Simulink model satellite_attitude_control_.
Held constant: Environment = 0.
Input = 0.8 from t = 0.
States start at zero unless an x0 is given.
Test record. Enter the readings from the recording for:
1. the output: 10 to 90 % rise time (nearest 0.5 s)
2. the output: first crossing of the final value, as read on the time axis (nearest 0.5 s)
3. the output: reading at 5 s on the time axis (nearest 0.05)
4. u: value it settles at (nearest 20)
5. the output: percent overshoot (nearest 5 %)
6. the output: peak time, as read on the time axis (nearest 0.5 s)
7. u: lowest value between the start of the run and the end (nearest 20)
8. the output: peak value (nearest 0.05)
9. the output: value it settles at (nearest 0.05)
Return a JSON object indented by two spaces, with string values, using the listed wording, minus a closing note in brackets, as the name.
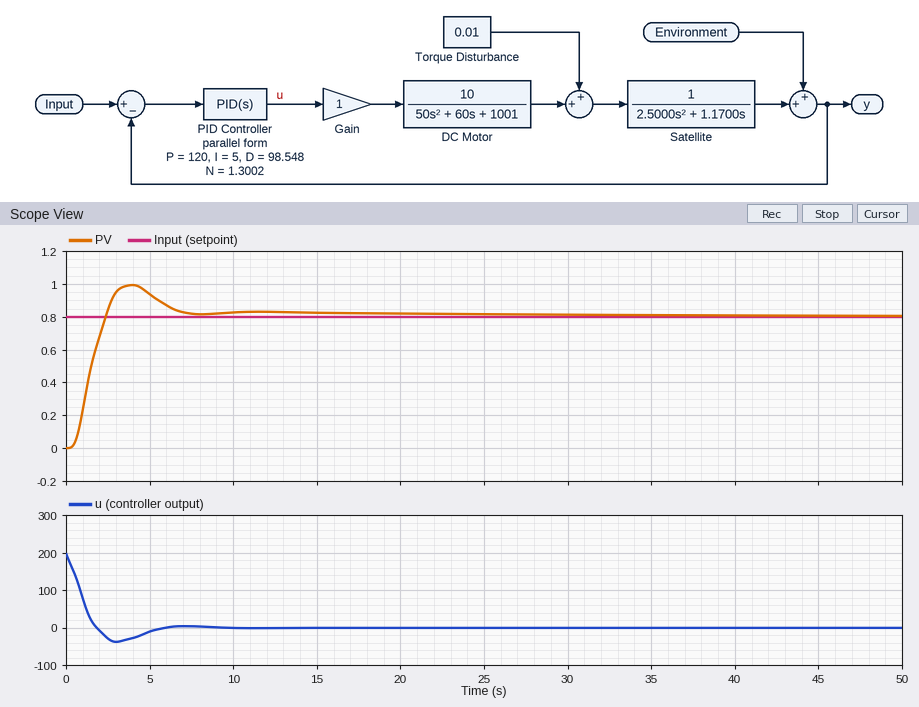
{
  "the output: 10 to 90 % rise time": "1.5 s",
  "the output: first crossing of the final value, as read on the time axis": "2.5 s",
  "the output: reading at 5 s on the time axis": "0.95",
  "u: value it settles at": "0",
  "the output: percent overshoot": "25 %",
  "the output: peak time, as read on the time axis": "4.0 s",
  "u: lowest value between the start of the run and the end": "-40",
  "the output: peak value": "1.00",
  "the output: value it settles at": "0.80"
}
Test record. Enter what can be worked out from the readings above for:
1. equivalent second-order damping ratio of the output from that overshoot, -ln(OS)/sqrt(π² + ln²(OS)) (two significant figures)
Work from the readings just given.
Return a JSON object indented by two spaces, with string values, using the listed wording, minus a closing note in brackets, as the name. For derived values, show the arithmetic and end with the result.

{
  "equivalent second-order damping ratio of the output from that overshoot, -ln(OS)/sqrt(π² + ln²(OS))": "ln(0.25) = -1.386; 1.386 / sqrt(9.870 + 1.922) = 0.40"
}
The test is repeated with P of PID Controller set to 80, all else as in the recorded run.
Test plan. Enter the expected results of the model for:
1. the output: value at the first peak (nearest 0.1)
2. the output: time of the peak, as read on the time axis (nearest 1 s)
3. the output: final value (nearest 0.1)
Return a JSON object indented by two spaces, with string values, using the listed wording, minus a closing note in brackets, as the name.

{
  "the output: value at the first peak": "0.9",
  "the output: time of the peak, as read on the time axis": "5 s",
  "the output: final value": "0.8"
}
